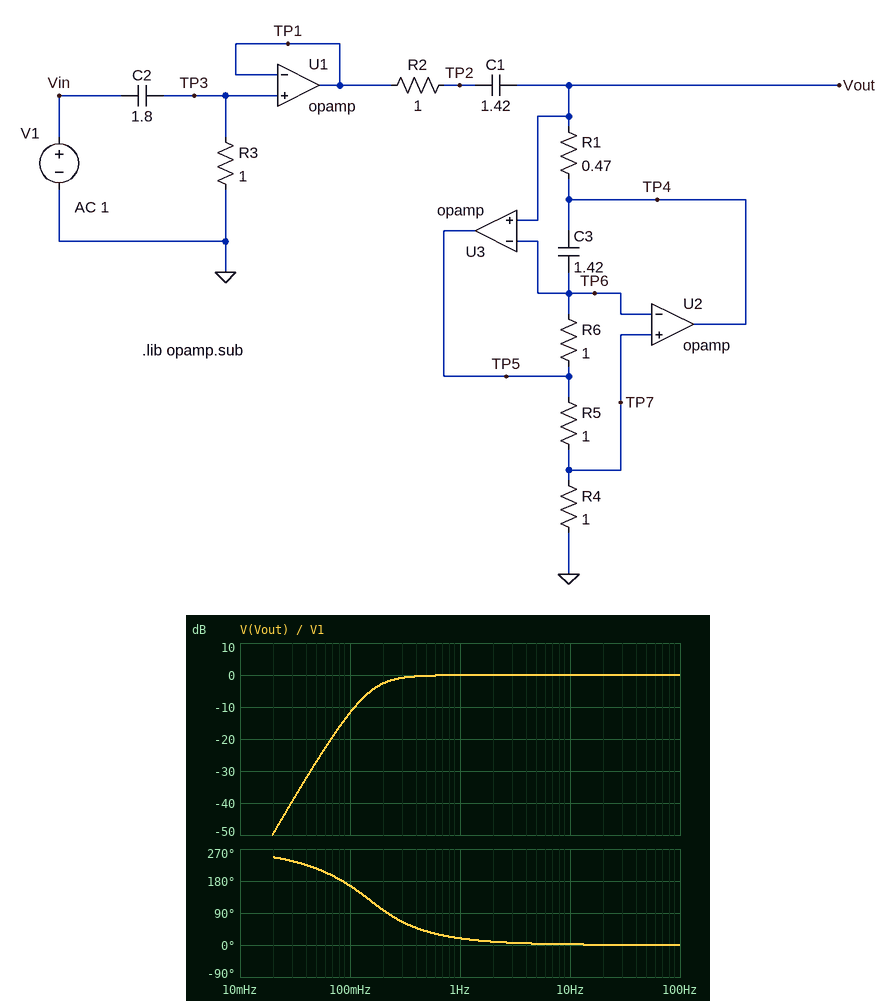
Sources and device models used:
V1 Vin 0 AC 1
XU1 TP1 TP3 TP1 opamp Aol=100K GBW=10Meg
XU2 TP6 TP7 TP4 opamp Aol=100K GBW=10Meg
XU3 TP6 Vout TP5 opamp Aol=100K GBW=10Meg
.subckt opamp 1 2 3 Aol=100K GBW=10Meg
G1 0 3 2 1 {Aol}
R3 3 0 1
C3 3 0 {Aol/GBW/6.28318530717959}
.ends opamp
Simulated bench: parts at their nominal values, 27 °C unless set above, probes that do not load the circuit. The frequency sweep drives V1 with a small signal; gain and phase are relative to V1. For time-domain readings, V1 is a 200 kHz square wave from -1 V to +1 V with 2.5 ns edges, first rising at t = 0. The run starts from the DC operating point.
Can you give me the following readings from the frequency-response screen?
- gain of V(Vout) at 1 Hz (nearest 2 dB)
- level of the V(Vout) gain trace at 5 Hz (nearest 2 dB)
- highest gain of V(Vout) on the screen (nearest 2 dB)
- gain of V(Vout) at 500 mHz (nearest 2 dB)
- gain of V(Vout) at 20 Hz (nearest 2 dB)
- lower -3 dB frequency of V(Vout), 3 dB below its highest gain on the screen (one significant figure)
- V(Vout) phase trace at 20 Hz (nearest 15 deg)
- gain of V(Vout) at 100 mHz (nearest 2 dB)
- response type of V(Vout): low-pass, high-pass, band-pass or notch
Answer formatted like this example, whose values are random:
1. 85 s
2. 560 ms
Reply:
1. 0 dB
2. 0 dB
3. 0 dB
4. 0 dB
5. 0 dB
6. 200 mHz
7. 0 deg
8. -12 dB
9. high-pass
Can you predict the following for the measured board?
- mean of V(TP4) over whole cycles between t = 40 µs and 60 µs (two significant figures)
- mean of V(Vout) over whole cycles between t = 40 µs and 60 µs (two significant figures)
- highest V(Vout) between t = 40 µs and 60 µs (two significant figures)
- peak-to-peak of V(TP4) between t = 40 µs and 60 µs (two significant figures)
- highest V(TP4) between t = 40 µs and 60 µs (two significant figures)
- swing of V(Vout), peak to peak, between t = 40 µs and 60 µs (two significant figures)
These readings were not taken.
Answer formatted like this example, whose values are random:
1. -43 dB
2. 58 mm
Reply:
1. 1.0 V
2. 1.0 V
3. 2.0 V
4. 2.0 V
5. 2.0 V
6. 2.0 V
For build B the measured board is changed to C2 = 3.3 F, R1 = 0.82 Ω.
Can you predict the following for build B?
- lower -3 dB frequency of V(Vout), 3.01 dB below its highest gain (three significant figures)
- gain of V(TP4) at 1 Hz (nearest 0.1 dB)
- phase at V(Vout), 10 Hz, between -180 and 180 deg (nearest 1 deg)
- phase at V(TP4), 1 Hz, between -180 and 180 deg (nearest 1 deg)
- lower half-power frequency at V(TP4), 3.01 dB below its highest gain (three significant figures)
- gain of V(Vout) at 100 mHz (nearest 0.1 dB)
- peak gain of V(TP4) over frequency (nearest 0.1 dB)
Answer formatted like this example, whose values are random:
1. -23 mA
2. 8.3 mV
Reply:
1. 113 mHz
2. 0.1 dB
3. 1 deg
4. 17 deg
5. 96.1 mHz
6. -4.2 dB
7. 1.9 dB
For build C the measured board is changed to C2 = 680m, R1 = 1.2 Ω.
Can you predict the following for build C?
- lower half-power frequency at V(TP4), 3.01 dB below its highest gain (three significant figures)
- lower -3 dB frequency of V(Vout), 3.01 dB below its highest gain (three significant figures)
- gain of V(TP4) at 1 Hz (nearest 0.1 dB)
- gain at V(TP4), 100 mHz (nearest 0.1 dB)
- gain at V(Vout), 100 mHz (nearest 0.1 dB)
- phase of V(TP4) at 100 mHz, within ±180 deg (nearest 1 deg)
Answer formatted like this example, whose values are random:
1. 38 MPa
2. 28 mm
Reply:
1. 110 mHz
2. 175 mHz
3. -0.1 dB
4. -4.0 dB
5. -7.5 dB
6. -152 deg
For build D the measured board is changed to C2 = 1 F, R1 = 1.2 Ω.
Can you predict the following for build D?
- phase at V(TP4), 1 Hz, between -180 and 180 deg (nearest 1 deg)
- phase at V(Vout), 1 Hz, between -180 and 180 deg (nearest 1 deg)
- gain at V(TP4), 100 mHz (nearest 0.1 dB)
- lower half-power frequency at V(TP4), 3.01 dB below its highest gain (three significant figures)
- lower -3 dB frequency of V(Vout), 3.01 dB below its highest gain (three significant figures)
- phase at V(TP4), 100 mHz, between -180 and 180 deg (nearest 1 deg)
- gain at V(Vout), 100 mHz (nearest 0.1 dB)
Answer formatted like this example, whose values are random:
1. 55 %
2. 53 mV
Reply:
1. 21 deg
2. 14 deg
3. -1.4 dB
4. 90.6 mHz
5. 116 mHz
6. -161 deg
7. -4.9 dB
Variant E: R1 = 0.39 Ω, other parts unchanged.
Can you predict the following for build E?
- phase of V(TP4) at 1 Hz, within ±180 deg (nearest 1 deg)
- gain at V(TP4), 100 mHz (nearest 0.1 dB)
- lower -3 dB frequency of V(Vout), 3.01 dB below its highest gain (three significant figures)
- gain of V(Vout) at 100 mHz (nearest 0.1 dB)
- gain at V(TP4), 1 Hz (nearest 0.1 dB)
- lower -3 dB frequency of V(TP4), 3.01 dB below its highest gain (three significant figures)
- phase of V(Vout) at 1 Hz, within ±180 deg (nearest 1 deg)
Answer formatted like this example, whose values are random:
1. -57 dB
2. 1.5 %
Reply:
1. 28 deg
2. -10.2 dB
3. 228 mHz
4. -13.7 dB
5. -0.1 dB
6. 194 mHz
7. 22 deg
